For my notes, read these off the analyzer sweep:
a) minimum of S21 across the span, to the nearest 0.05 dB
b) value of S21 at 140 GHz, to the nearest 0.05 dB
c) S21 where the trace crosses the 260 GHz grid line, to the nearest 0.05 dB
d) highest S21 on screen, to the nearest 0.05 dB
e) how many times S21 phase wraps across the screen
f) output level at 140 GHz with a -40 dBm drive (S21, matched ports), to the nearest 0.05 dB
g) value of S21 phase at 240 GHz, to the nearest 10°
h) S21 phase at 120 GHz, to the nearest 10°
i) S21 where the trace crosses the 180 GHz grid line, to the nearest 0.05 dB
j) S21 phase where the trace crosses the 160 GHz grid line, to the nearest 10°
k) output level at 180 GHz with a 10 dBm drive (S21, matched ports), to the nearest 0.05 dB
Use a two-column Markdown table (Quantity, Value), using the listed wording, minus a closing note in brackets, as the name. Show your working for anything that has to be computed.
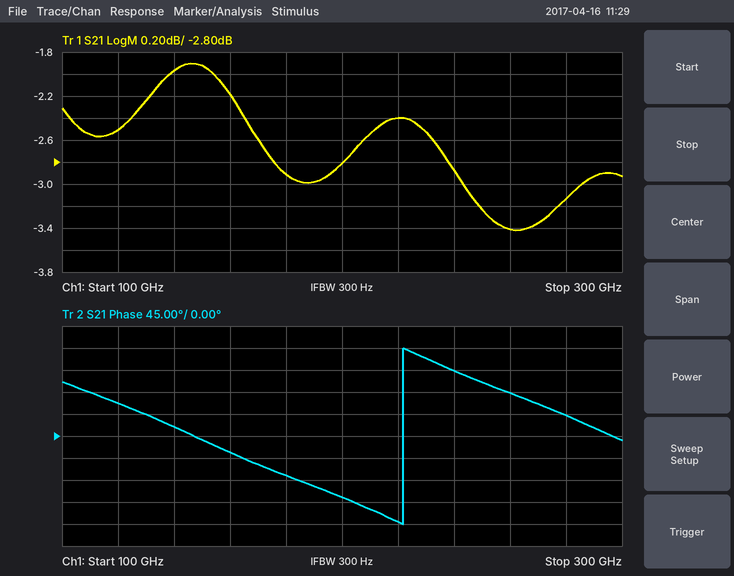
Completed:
| Quantity | Value |
|---|---|
| minimum of S21 across the span, to the nearest 0.05 dB | -3.40 dB |
| value of S21 at 140 GHz, to the nearest 0.05 dB | -1.95 dB |
| S21 where the trace crosses the 260 GHz grid line, to the nearest 0.05 dB | -3.40 dB |
| highest S21 on screen, to the nearest 0.05 dB | -1.90 dB |
| how many times S21 phase wraps across the screen | 1 |
| output level at 140 GHz with a -40 dBm drive (S21, matched ports), to the nearest 0.05 dB | -40 dBm + (-1.95 dB) = -41.95 dBm |
| value of S21 phase at 240 GHz, to the nearest 10° | 130° |
| S21 phase at 120 GHz, to the nearest 10° | 70° |
| S21 where the trace crosses the 180 GHz grid line, to the nearest 0.05 dB | -2.90 dB |
| S21 phase where the trace crosses the 160 GHz grid line, to the nearest 10° | -30° |
| output level at 180 GHz with a 10 dBm drive (S21, matched ports), to the nearest 0.05 dB | 10 dBm + (-2.90 dB) = 7.10 dBm |
